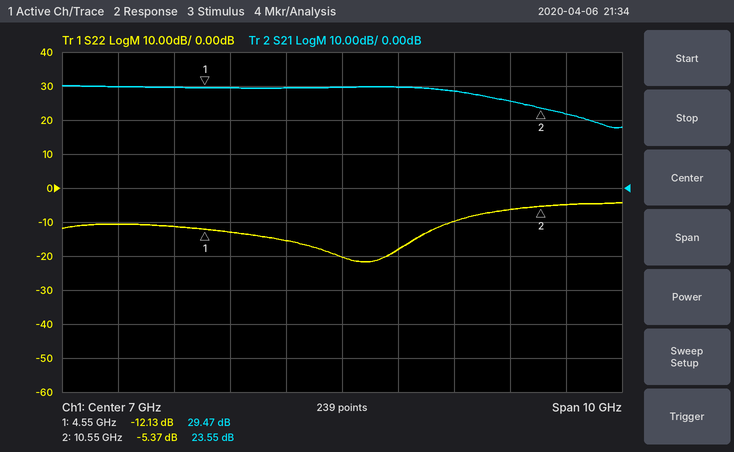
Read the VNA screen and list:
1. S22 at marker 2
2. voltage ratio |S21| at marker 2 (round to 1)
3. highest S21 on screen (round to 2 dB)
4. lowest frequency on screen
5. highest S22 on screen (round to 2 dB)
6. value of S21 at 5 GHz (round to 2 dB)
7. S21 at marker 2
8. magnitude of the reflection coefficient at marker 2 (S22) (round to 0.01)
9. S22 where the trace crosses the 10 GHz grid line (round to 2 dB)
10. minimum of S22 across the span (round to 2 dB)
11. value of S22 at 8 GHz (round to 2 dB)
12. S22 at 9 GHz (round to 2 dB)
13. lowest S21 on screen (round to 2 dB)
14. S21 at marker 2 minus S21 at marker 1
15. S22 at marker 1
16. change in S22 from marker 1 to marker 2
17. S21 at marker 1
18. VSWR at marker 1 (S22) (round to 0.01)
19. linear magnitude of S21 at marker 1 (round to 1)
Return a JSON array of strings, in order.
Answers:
["-5.37 dB", "15", "30 dB", "2 GHz", "-4 dB", "30 dB", "23.55 dB", "0.54", "-6 dB", "-22 dB", "-18 dB", "-10 dB", "18 dB", "-5.92 dB", "-12.13 dB", "6.76 dB", "29.47 dB", "1.66", "30"]
